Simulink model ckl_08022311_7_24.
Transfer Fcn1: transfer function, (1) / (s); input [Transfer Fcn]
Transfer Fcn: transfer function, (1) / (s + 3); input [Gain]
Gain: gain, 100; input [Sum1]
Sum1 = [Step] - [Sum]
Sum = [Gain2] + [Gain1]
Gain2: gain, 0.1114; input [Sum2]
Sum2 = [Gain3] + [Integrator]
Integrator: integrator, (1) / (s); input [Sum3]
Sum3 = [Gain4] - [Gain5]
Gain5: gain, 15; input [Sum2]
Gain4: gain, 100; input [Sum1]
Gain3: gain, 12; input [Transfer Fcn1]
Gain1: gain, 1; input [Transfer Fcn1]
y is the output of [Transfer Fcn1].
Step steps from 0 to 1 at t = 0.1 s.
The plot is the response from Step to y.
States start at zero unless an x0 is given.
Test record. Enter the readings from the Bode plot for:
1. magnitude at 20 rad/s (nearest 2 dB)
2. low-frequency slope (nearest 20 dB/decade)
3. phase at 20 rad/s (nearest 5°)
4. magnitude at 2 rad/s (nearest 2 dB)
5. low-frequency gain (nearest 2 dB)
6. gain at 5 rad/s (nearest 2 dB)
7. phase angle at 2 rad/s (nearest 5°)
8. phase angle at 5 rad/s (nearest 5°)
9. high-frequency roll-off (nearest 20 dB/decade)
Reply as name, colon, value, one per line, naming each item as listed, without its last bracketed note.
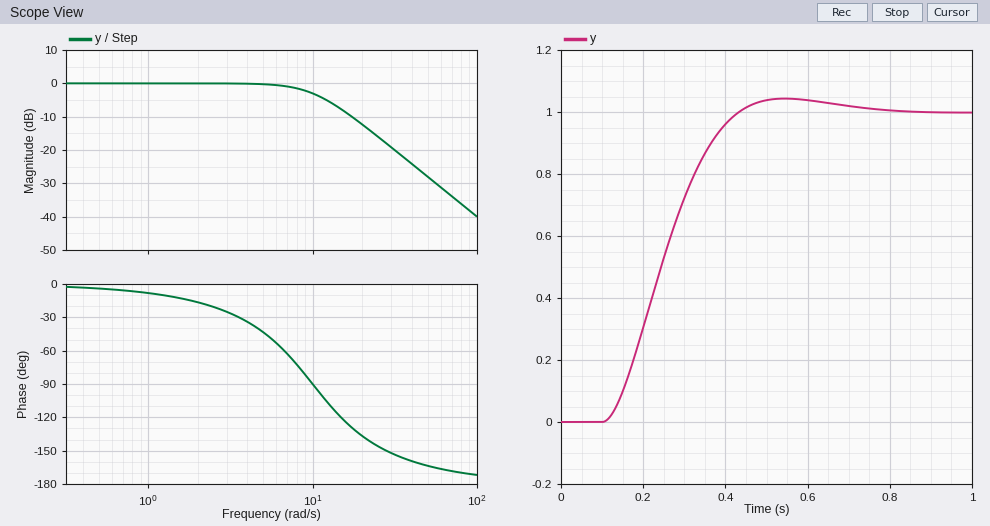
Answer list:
magnitude at 20 rad/s: -12 dB
low-frequency slope: 0 dB/decade
phase at 20 rad/s: -135°
magnitude at 2 rad/s: 0 dB
low-frequency gain: 0 dB
gain at 5 rad/s: 0 dB
phase angle at 2 rad/s: -15°
phase angle at 5 rad/s: -45°
high-frequency roll-off: -40 dB/decade
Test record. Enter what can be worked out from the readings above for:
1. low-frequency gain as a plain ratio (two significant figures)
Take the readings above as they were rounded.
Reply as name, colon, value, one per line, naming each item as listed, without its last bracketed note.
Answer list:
low-frequency gain as a plain ratio: 1.0
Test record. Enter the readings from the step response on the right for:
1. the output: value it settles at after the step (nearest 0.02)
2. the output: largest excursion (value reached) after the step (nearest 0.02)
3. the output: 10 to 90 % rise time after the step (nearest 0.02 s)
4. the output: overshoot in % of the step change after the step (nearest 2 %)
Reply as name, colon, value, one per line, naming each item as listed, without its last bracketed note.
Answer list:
the output: value it settles at after the step: 1.00
the output: largest excursion (value reached) after the step: 1.04
the output: 10 to 90 % rise time after the step: 0.22 s
the output: overshoot in % of the step change after the step: 4 %
